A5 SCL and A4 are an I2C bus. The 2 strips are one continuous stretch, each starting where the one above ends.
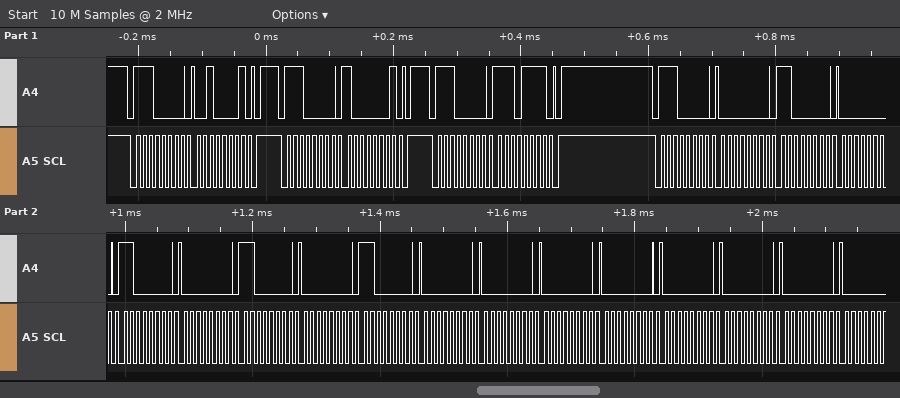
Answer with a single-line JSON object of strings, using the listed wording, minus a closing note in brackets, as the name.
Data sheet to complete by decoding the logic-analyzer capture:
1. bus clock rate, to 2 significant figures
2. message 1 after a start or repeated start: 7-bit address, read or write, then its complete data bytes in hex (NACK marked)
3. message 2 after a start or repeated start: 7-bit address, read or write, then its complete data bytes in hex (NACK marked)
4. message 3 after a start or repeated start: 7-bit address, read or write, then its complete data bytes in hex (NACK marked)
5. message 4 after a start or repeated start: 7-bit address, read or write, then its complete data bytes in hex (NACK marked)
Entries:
{"bus clock rate, to 2 significant figures": "100 kHz", "message 1 after a start or repeated start: 7-bit address, read or write, then its complete data bytes in hex": "0x70 write: 21", "message 2 after a start or repeated start: 7-bit address, read or write, then its complete data bytes in hex": "0x70 write: 81", "message 3 after a start or repeated start: 7-bit address, read or write, then its complete data bytes in hex": "0x70 write: EF", "message 4 after a start or repeated start: 7-bit address, read or write, then its complete data bytes in hex": "0x70 write: 00 C0 00 C0 00 C0 00 C0 00 00 00 00 00 00 00"}
